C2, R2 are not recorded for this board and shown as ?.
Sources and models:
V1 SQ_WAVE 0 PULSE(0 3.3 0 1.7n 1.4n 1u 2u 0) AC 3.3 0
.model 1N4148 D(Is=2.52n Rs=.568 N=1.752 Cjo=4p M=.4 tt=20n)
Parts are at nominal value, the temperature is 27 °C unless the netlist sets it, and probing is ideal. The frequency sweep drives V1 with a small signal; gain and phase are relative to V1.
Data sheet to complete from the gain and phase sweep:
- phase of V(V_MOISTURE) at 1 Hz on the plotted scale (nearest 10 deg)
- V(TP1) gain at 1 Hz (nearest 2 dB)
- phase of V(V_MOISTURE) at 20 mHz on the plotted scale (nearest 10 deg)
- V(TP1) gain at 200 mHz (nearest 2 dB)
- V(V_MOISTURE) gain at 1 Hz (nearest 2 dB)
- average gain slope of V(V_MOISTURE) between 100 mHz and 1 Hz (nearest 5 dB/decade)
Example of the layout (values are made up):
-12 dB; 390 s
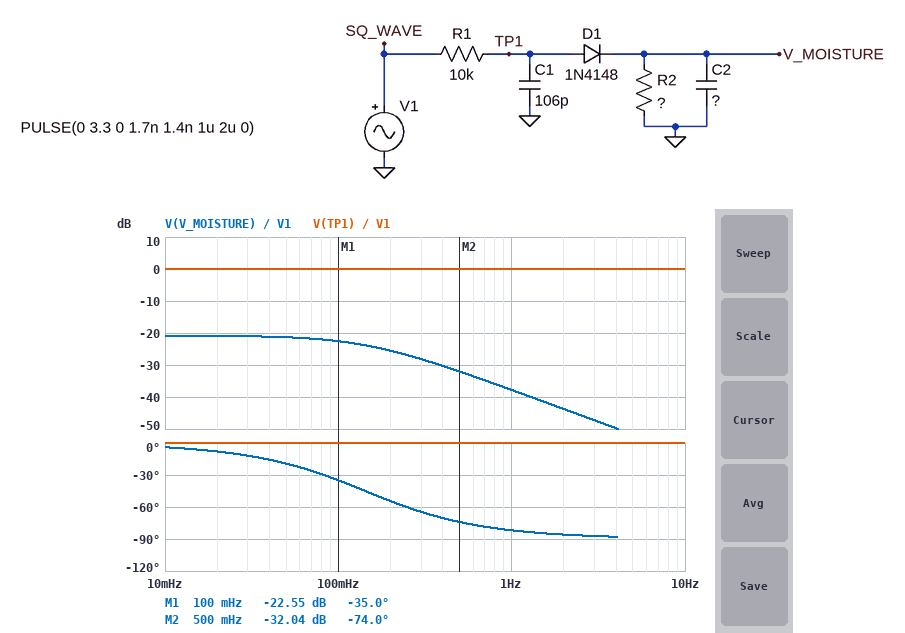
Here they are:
-80 deg; 0 dB; -10 deg; 0 dB; -38 dB; -15 dB/decade
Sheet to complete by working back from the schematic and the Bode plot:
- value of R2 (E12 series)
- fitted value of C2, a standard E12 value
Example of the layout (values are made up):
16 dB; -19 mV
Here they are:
1.8 MΩ; 680 nF
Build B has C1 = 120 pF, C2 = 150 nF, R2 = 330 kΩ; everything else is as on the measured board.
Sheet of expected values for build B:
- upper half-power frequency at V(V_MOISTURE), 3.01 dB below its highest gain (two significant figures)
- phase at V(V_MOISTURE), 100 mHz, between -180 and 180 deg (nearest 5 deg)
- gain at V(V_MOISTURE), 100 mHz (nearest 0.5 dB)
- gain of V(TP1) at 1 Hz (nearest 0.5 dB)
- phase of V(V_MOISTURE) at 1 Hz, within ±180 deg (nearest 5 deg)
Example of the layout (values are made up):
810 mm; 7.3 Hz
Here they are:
3.3 Hz; 0 deg; -35.0 dB; 0 dB; -15 deg
